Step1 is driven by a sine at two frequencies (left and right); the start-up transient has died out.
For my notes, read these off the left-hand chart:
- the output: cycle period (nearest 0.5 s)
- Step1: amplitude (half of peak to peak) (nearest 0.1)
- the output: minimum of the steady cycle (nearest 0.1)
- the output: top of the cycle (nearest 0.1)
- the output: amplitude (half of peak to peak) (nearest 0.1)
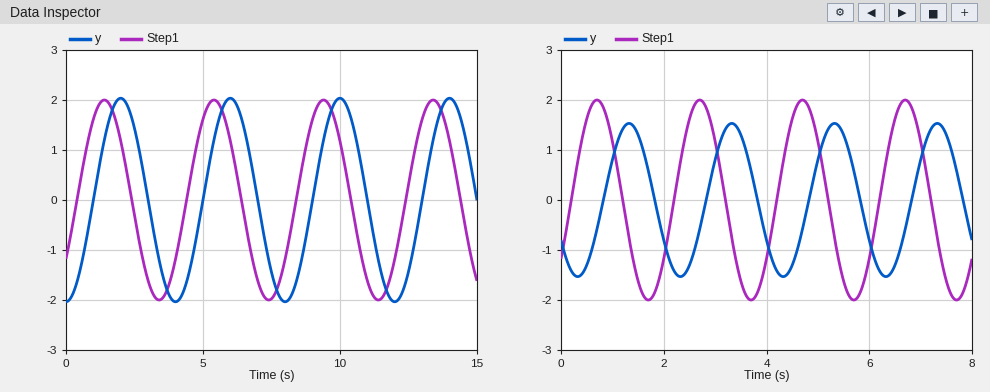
4.0 s
2.0
-2.0
2.0
2.0
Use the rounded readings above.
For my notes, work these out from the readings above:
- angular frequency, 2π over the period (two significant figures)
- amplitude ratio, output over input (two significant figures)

1.6 rad/s
1.0
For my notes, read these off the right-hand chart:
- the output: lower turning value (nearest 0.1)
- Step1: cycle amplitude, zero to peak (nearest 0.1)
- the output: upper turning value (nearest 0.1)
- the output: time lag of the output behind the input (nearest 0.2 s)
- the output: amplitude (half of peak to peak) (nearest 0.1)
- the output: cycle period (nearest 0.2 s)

-1.5
2.0
1.5
0.6 s
1.5
2.0 s
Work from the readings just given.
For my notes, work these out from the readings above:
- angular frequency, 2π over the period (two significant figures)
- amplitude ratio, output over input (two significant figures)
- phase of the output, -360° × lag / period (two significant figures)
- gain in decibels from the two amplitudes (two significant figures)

3.1 rad/s
0.75
-110°
-2.5 dB
